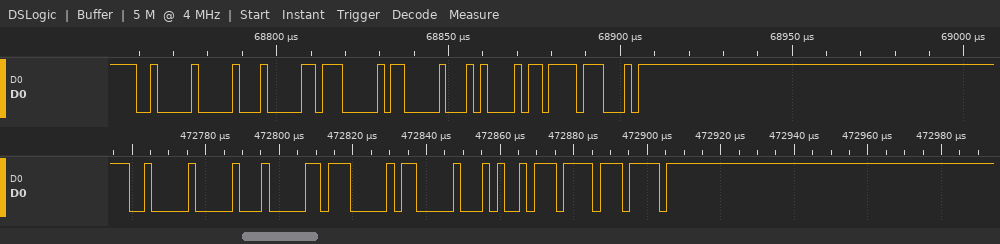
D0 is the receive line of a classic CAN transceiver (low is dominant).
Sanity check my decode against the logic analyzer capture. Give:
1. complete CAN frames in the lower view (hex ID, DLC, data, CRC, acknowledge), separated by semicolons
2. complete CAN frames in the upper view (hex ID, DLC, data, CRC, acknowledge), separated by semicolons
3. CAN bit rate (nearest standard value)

ID 200, DLC 4, data 17 03 00 A5, CRC 6F77, ACK
ID 200, DLC 4, data 17 03 00 A1, CRC 37B8, ACK
500 kbit/s
